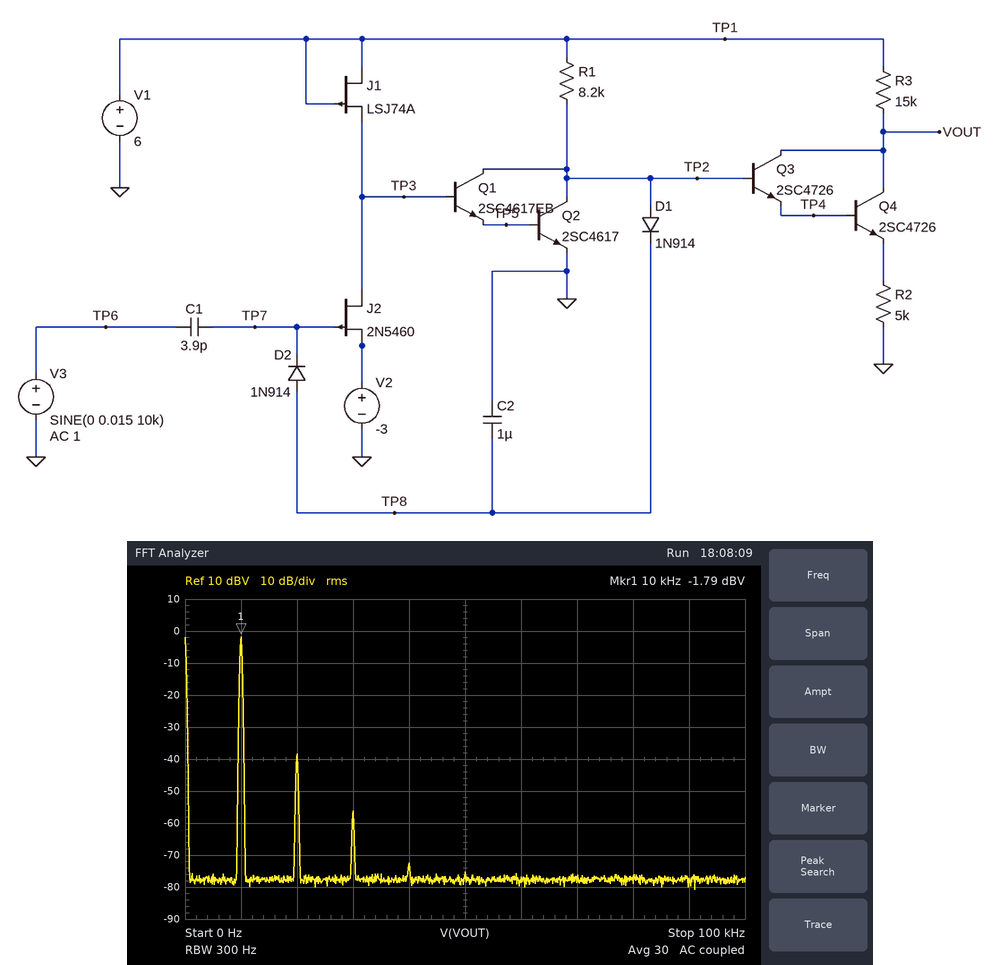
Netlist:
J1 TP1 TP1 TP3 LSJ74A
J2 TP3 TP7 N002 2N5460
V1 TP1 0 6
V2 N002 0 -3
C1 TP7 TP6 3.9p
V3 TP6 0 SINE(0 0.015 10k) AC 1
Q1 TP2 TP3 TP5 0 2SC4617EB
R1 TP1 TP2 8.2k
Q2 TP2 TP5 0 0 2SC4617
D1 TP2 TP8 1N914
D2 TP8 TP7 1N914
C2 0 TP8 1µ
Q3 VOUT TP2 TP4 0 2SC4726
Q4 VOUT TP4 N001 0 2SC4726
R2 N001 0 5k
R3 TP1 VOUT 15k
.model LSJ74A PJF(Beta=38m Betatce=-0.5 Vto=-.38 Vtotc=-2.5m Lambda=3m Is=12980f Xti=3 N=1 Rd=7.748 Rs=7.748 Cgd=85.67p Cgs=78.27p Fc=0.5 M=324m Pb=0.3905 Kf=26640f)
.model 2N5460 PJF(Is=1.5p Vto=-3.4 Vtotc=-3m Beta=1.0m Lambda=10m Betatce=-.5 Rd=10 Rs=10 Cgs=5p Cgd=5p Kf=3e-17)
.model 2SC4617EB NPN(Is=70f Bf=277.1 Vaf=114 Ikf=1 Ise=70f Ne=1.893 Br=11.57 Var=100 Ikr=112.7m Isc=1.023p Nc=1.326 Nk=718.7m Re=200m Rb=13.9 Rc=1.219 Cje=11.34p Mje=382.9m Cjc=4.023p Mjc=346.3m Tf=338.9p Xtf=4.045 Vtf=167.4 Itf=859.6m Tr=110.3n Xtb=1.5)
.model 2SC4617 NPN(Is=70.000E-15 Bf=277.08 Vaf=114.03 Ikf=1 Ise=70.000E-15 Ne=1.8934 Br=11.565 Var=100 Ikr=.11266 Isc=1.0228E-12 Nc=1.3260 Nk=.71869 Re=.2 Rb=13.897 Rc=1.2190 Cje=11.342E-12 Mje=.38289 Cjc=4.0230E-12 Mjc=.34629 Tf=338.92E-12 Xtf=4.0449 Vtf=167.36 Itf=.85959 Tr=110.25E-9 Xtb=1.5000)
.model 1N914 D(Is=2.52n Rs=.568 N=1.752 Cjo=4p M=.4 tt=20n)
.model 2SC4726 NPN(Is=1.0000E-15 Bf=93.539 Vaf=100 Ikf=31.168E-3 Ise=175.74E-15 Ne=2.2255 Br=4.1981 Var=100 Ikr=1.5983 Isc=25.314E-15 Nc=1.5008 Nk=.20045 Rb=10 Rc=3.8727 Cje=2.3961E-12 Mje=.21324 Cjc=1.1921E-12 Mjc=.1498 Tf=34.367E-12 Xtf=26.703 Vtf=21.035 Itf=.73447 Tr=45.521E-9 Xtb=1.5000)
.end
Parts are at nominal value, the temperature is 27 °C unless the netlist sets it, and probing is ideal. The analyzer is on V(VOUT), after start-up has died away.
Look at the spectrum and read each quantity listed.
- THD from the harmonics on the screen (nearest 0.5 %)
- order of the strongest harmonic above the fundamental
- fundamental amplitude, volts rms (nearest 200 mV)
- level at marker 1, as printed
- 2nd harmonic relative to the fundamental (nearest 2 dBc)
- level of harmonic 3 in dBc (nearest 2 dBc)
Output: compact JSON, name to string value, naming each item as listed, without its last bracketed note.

{"THD from the harmonics on the screen": "1.5 %", "order of the strongest harmonic above the fundamental": "2", "fundamental amplitude, volts rms": "800 mV", "level at marker 1, as printed": "-1.79 dBV", "2nd harmonic relative to the fundamental": "-36 dBc", "level of harmonic 3 in dBc": "-54 dBc"}
